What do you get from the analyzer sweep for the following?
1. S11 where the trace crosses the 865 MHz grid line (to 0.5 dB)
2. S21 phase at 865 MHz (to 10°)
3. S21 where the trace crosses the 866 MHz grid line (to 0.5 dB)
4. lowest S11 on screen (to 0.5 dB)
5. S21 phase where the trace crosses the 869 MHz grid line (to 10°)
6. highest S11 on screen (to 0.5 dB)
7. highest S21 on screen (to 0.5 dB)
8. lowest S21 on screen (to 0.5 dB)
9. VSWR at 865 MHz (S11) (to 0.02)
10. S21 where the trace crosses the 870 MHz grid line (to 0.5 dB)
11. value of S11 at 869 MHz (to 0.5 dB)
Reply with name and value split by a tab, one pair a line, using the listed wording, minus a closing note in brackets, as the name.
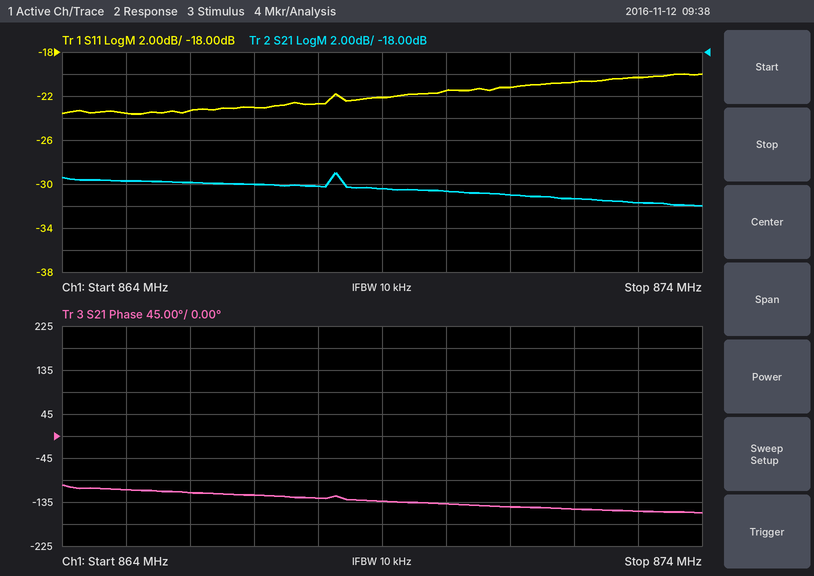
S11 where the trace crosses the 865 MHz grid line	-23.5 dB
S21 phase at 865 MHz	-110°
S21 where the trace crosses the 866 MHz grid line	-30.0 dB
lowest S11 on screen	-23.5 dB
S21 phase where the trace crosses the 869 MHz grid line	-130°
highest S11 on screen	-20.0 dB
highest S21 on screen	-29.0 dB
lowest S21 on screen	-32.0 dB
VSWR at 865 MHz (S11)	1.14
S21 where the trace crosses the 870 MHz grid line	-30.5 dB
value of S11 at 869 MHz	-22.0 dB
